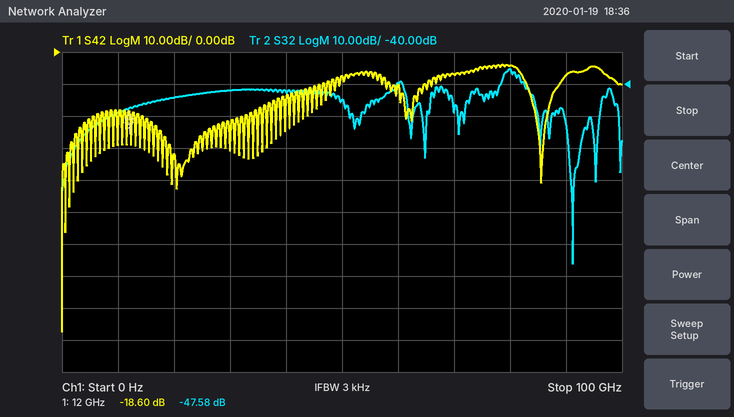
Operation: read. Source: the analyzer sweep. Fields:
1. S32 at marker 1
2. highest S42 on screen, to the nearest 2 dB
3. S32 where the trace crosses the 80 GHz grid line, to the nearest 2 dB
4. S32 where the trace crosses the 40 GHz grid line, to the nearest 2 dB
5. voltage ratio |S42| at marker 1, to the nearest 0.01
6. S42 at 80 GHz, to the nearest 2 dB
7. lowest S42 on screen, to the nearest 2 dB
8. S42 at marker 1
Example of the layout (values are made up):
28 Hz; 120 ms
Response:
-47.58 dB; -4 dB; -36 dB; -42 dB; 0.12; -4 dB; -88 dB; -18.60 dB
